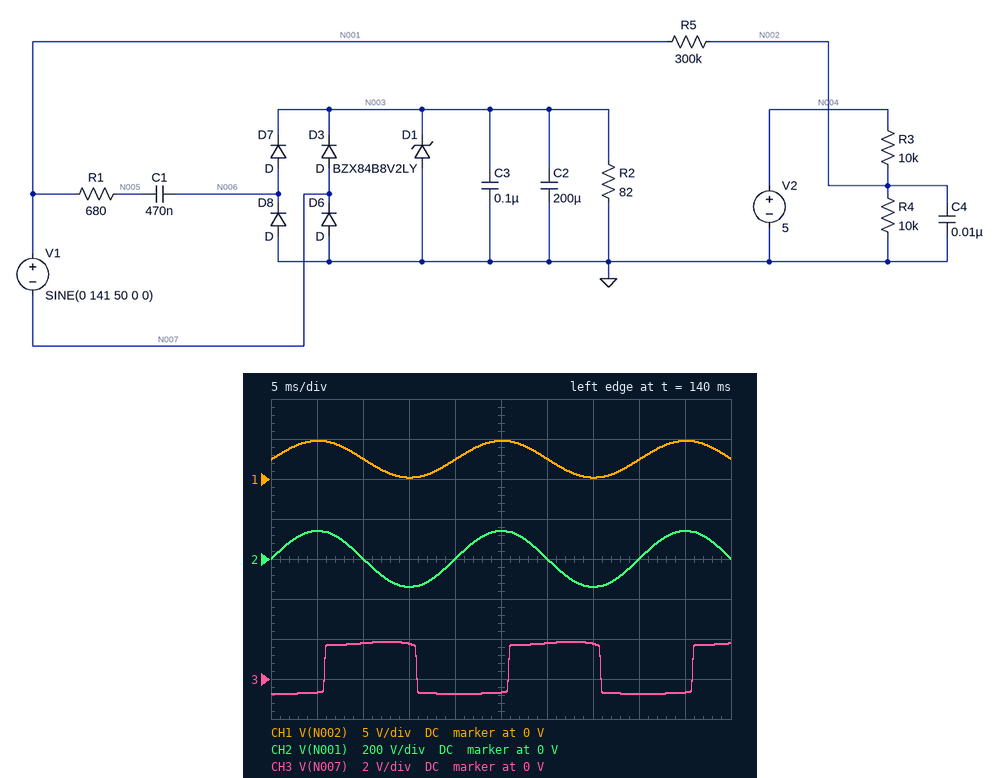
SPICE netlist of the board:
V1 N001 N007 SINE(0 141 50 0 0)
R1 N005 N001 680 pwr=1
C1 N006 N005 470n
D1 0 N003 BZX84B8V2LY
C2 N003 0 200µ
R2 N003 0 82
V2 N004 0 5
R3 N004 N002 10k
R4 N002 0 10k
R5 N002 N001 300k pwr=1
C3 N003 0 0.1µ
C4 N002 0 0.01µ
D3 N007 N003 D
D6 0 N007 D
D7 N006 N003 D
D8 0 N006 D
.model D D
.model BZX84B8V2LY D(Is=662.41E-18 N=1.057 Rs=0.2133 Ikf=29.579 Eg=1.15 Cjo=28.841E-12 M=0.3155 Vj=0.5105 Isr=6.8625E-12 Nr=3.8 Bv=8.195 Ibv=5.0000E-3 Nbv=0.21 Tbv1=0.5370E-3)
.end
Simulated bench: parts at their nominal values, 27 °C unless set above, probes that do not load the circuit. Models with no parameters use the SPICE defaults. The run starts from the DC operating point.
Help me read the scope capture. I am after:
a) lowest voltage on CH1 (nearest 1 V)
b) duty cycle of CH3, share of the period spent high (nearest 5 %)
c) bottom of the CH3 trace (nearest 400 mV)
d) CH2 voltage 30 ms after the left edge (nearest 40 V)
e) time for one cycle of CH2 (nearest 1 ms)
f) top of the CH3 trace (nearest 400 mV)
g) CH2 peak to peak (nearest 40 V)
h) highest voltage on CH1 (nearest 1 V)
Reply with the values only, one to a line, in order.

0 V
50 %
-800 mV
0 V
20 ms
2.0 V
280 V
5 V
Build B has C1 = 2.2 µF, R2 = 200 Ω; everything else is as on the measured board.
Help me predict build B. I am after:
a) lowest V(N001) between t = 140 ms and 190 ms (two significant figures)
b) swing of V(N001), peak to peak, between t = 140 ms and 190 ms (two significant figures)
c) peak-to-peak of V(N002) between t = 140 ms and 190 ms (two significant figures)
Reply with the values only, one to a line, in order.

-130 V
270 V
4.5 V
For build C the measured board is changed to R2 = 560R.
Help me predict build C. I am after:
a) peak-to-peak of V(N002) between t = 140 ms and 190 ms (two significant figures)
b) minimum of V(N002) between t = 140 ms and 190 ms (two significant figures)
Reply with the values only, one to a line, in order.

4.5 V
250 mV
